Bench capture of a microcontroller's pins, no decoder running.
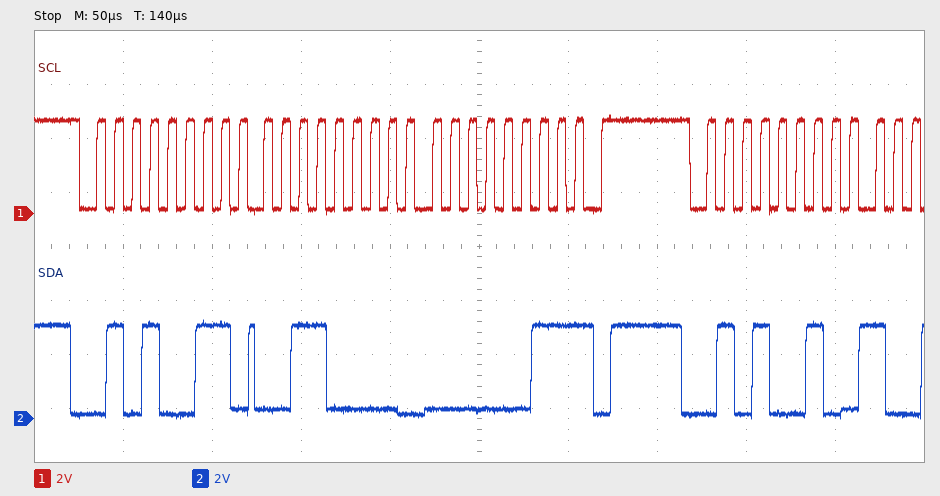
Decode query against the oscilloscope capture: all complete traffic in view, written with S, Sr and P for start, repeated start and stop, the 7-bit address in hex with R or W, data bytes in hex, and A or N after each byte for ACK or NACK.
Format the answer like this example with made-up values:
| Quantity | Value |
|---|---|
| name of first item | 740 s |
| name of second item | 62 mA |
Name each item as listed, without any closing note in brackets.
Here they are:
| Quantity | Value |
|---|---|
| all complete traffic in view, written with S, Sr and P for start, repeated start and stop, the 7-bit address in hex with R or W, data bytes in hex, and A or N after each byte for ACK or NACK | S 29R A 30 A 03 N P S 29W A |
